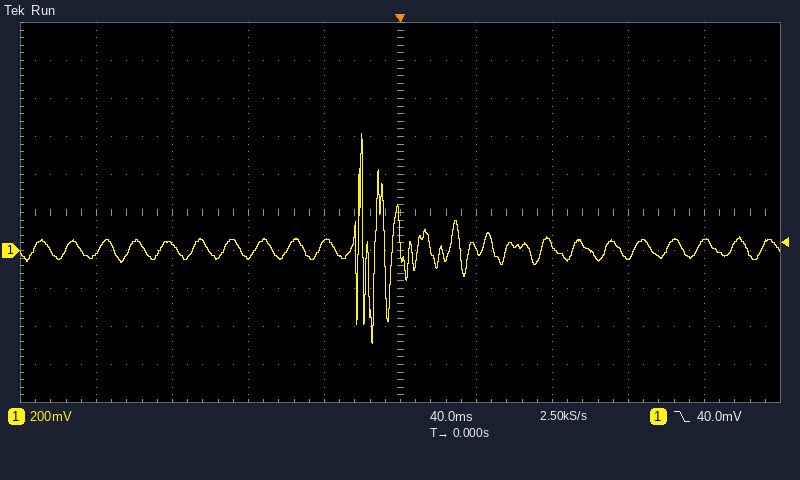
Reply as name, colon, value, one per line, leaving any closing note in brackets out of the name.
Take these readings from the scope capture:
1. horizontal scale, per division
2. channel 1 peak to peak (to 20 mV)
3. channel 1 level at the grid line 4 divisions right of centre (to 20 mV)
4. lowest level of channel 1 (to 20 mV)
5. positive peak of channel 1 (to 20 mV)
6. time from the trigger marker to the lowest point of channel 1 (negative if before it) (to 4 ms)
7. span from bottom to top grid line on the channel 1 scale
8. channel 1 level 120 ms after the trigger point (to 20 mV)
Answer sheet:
horizontal scale, per division: 40 ms
channel 1 peak to peak: 1.10 V
channel 1 level at the grid line 4 divisions right of centre: 40 mV
lowest level of channel 1: -480 mV
positive peak of channel 1: 620 mV
time from the trigger marker to the lowest point of channel 1 (negative if before it): -16 ms
span from bottom to top grid line on the channel 1 scale: 2 V
channel 1 level 120 ms after the trigger point: -40 mV
